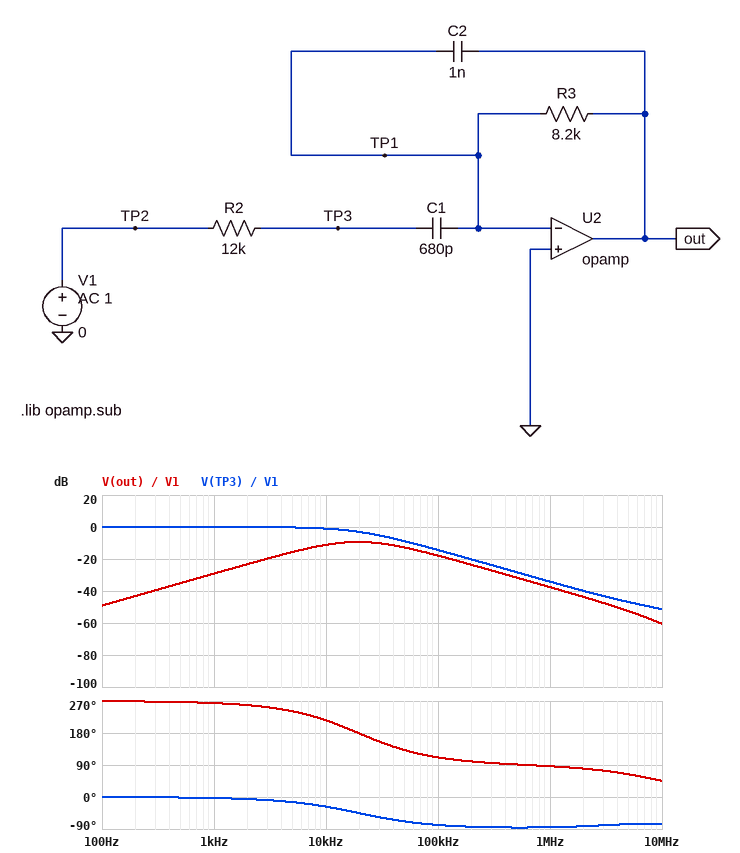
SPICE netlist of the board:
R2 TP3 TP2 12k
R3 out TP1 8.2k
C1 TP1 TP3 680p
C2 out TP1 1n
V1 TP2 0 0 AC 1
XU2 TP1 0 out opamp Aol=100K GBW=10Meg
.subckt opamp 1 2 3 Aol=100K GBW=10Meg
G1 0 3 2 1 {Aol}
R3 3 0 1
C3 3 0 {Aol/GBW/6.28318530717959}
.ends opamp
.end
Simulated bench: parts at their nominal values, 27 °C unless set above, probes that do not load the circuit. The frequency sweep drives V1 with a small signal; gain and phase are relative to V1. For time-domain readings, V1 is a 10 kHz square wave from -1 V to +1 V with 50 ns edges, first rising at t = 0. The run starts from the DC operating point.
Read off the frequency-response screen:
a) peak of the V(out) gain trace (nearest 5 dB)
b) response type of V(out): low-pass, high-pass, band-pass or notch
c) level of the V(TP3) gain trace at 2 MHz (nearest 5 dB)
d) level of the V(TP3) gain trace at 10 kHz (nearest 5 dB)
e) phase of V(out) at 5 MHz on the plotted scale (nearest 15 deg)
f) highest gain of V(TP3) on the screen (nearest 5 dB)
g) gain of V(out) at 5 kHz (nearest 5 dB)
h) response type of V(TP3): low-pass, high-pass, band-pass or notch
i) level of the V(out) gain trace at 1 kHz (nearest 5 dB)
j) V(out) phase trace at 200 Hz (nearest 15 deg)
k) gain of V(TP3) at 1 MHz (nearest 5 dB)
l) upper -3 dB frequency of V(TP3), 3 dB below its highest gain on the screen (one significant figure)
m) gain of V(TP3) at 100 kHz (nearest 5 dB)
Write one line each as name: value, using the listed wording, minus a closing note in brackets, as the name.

peak of the V(out) gain trace: -10 dB
response type of V(out): low-pass, high-pass, band-pass or notch: band-pass
level of the V(TP3) gain trace at 2 MHz: -40 dB
level of the V(TP3) gain trace at 10 kHz: 0 dB
phase of V(out) at 5 MHz on the plotted scale: 60 deg
highest gain of V(TP3) on the screen: 0 dB
gain of V(out) at 5 kHz: -15 dB
response type of V(TP3): low-pass, high-pass, band-pass or notch: low-pass
level of the V(out) gain trace at 1 kHz: -30 dB
V(out) phase trace at 200 Hz: 270 deg
gain of V(TP3) at 1 MHz: -35 dB
upper -3 dB frequency of V(TP3), 3 dB below its highest gain on the screen: 20 kHz
gain of V(TP3) at 100 kHz: -15 dB
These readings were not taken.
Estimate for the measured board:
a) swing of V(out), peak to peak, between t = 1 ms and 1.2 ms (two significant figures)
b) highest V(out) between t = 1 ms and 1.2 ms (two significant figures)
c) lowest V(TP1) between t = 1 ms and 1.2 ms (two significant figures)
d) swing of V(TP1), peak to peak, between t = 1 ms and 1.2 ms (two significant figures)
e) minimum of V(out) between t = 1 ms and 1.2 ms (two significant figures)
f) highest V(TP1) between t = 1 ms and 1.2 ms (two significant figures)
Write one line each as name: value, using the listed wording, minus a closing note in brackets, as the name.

swing of V(out), peak to peak, between t = 1 ms and 1.2 ms: 990 mV
highest V(out) between t = 1 ms and 1.2 ms: 490 mV
lowest V(TP1) between t = 1 ms and 1.2 ms: -2.6 mV
swing of V(TP1), peak to peak, between t = 1 ms and 1.2 ms: 5.3 mV
minimum of V(out) between t = 1 ms and 1.2 ms: -490 mV
highest V(TP1) between t = 1 ms and 1.2 ms: 2.6 mV
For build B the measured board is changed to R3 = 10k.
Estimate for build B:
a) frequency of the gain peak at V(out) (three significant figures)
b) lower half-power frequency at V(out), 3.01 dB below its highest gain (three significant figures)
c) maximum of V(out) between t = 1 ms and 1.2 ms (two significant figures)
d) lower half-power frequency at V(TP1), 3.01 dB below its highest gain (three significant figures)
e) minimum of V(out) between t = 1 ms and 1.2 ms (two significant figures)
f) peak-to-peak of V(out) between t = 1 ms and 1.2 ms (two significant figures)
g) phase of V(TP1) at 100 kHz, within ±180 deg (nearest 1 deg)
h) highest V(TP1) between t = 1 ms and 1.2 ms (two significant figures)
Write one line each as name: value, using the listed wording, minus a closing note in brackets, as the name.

frequency of the gain peak at V(out): 17.6 kHz
lower half-power frequency at V(out), 3.01 dB below its highest gain: 7.27 kHz
maximum of V(out) between t = 1 ms and 1.2 ms: 540 mV
lower half-power frequency at V(TP1), 3.01 dB below its highest gain: 27.4 kHz
minimum of V(out) between t = 1 ms and 1.2 ms: -540 mV
peak-to-peak of V(out) between t = 1 ms and 1.2 ms: 1.1 V
phase of V(TP1) at 100 kHz, within ±180 deg: 19 deg
highest V(TP1) between t = 1 ms and 1.2 ms: 2.7 mV
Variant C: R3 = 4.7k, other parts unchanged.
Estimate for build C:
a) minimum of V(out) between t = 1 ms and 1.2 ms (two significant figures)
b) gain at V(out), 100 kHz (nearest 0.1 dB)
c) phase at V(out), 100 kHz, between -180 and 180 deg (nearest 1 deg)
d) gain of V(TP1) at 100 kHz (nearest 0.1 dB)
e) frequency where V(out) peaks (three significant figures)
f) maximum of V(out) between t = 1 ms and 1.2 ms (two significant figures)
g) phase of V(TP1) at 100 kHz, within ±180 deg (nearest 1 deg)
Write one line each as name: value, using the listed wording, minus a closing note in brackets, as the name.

minimum of V(out) between t = 1 ms and 1.2 ms: -370 mV
gain at V(out), 100 kHz: -18.2 dB
phase at V(out), 100 kHz, between -180 and 180 deg: 119 deg
gain of V(TP1) at 100 kHz: -58.2 dB
frequency where V(out) peaks: 25.7 kHz
maximum of V(out) between t = 1 ms and 1.2 ms: 370 mV
phase of V(TP1) at 100 kHz, within ±180 deg: 29 deg
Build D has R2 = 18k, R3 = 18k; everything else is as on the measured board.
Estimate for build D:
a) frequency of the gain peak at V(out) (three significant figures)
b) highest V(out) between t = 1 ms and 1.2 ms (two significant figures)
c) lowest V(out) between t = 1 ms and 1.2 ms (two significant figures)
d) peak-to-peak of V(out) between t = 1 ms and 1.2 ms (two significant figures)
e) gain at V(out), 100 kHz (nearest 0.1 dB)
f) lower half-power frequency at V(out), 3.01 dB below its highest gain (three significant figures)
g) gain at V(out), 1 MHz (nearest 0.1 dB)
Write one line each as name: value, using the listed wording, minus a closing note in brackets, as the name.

frequency of the gain peak at V(out): 10.7 kHz
highest V(out) between t = 1 ms and 1.2 ms: 510 mV
lowest V(out) between t = 1 ms and 1.2 ms: -510 mV
peak-to-peak of V(out) between t = 1 ms and 1.2 ms: 1.0 V
gain at V(out), 100 kHz: -21.2 dB
lower half-power frequency at V(out), 3.01 dB below its highest gain: 4.38 kHz
gain at V(out), 1 MHz: -41.1 dB
